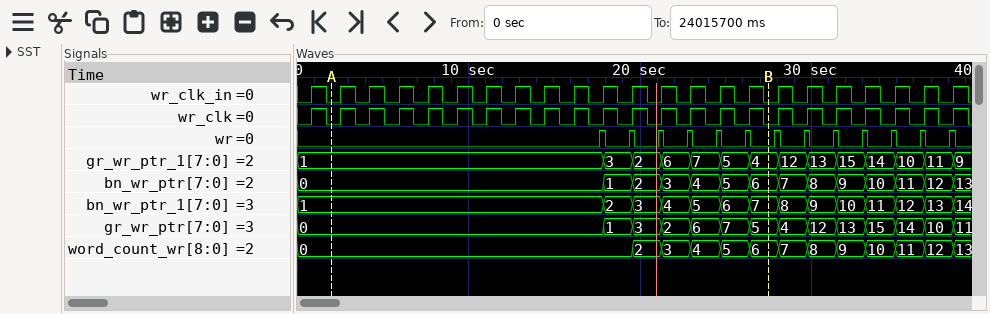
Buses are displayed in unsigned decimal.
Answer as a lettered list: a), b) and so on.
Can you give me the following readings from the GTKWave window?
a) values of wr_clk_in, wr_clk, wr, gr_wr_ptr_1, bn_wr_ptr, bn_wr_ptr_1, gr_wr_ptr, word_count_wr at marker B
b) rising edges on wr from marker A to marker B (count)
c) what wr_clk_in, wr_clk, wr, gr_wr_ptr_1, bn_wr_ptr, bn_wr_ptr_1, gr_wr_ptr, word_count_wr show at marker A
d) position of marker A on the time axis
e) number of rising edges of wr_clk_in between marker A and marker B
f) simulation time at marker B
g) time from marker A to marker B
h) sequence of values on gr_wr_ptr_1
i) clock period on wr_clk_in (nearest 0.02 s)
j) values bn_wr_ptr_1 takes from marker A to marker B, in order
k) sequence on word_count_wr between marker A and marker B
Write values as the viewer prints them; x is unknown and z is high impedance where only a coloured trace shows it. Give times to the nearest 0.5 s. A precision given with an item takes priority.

a) wr_clk_in=0, wr_clk=0, wr=0, gr_wr_ptr_1=4, bn_wr_ptr=6, bn_wr_ptr_1=7, gr_wr_ptr=5, word_count_wr=6
b) 6
c) wr_clk_in=0, wr_clk=0, wr=0, gr_wr_ptr_1=1, bn_wr_ptr=0, bn_wr_ptr_1=1, gr_wr_ptr=0, word_count_wr=0
d) 2 s
e) 15
f) 27.5 s
g) 25.5 s
h) 1, 3, 2, 6, 7, 5, 4, 12, 13, 15, 14, 10, 11, 9
i) 1.7 s
j) 1, 2, 3, 4, 5, 6, 7
k) 0, 2, 3, 4, 5, 6
